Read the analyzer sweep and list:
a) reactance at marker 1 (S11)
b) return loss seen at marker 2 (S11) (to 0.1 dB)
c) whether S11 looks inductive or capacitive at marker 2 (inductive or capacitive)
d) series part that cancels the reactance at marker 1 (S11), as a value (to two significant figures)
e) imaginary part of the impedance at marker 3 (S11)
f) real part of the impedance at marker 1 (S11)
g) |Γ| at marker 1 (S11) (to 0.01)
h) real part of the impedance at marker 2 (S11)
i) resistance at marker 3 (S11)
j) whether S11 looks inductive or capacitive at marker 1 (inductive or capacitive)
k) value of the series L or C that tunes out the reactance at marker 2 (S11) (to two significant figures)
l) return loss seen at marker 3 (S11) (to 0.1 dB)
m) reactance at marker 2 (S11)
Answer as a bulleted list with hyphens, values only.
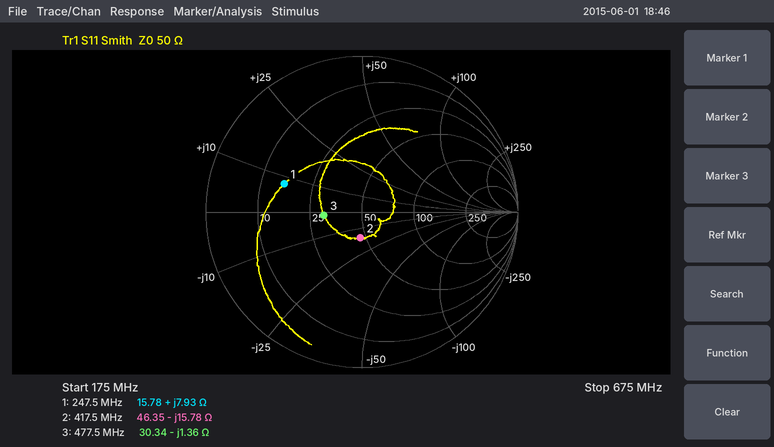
- +7.93 Ω
- 15.6 dB
- capacitive
- 81 pF
- -1.36 Ω
- 15.78 Ω
- 0.53
- 46.35 Ω
- 30.34 Ω
- inductive
- 6.0 nH
- 12.2 dB
- -15.78 Ω
